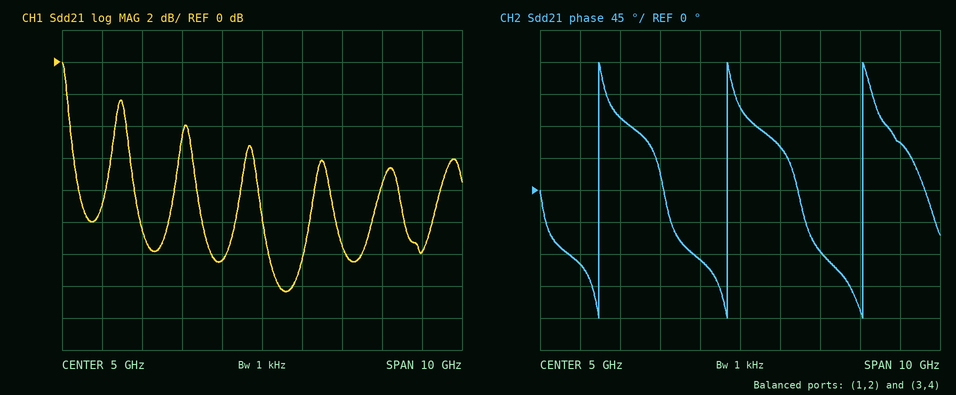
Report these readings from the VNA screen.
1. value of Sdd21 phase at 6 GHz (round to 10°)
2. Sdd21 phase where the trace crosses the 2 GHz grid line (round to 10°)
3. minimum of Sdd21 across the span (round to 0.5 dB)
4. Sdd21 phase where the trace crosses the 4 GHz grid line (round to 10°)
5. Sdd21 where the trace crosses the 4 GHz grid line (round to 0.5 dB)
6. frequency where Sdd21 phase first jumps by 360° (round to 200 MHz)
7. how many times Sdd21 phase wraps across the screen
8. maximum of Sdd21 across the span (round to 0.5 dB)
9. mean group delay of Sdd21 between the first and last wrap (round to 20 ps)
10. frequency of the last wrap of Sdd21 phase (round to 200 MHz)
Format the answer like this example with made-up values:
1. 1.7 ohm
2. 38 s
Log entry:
1. 60°
2. 100°
3. -14.5 dB
4. -100°
5. -12.5 dB
6. 1.4 GHz
7. 3
8. 0.0 dB
9. 300 ps
10. 8.0 GHz
